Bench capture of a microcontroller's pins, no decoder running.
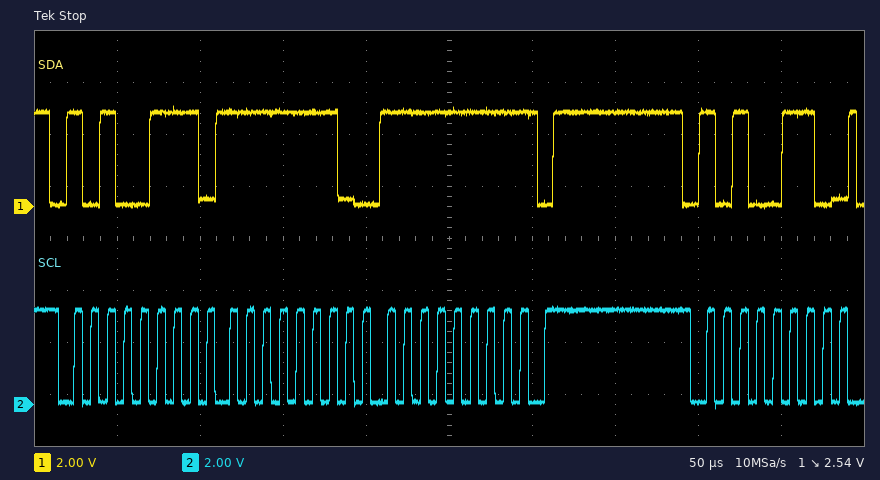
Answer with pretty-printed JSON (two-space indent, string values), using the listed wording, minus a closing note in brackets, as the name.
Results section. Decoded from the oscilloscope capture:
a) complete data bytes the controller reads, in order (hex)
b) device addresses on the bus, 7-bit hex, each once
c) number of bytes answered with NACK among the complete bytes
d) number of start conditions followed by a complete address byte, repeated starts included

{
  "complete data bytes the controller reads, in order": "FE FF",
  "device addresses on the bus, 7-bit hex, each once": "0x53",
  "number of bytes answered with NACK among the complete bytes": "1",
  "number of start conditions followed by a complete address byte, repeated starts included": "2"
}
